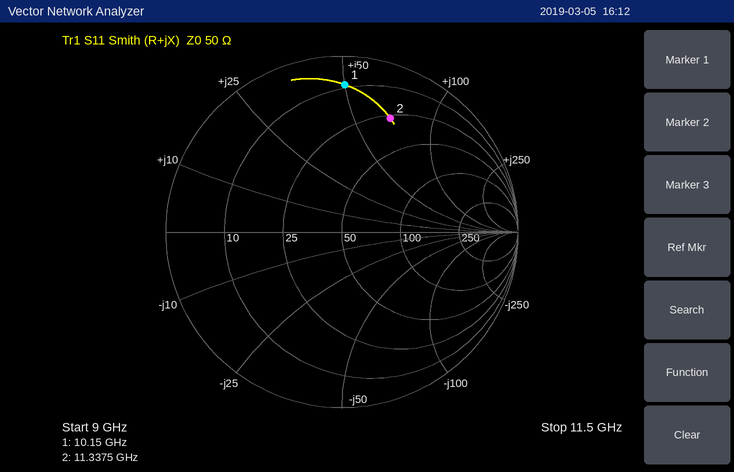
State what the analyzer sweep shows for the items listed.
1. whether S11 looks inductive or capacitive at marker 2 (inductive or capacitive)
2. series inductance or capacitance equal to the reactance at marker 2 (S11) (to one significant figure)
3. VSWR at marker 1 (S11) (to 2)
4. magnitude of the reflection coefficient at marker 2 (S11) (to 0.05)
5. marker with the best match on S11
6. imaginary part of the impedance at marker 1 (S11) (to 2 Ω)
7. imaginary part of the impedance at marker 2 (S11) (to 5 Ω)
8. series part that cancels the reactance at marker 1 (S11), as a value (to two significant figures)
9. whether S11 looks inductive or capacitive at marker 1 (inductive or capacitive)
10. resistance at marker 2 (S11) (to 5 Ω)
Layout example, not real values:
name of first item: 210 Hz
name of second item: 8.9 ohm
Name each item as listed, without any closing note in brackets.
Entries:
whether S11 looks inductive or capacitive at marker 2: inductive
series inductance or capacitance equal to the reactance at marker 2 (S11): 1.0 nH
VSWR at marker 1 (S11): 12
magnitude of the reflection coefficient at marker 2 (S11): 0.70
marker with the best match on S11: marker 2
imaginary part of the impedance at marker 1 (S11): +50 Ω
imaginary part of the impedance at marker 2 (S11): +70 Ω
series part that cancels the reactance at marker 1 (S11), as a value: 310 fF
whether S11 looks inductive or capacitive at marker 1: inductive
resistance at marker 2 (S11): 25 Ω
